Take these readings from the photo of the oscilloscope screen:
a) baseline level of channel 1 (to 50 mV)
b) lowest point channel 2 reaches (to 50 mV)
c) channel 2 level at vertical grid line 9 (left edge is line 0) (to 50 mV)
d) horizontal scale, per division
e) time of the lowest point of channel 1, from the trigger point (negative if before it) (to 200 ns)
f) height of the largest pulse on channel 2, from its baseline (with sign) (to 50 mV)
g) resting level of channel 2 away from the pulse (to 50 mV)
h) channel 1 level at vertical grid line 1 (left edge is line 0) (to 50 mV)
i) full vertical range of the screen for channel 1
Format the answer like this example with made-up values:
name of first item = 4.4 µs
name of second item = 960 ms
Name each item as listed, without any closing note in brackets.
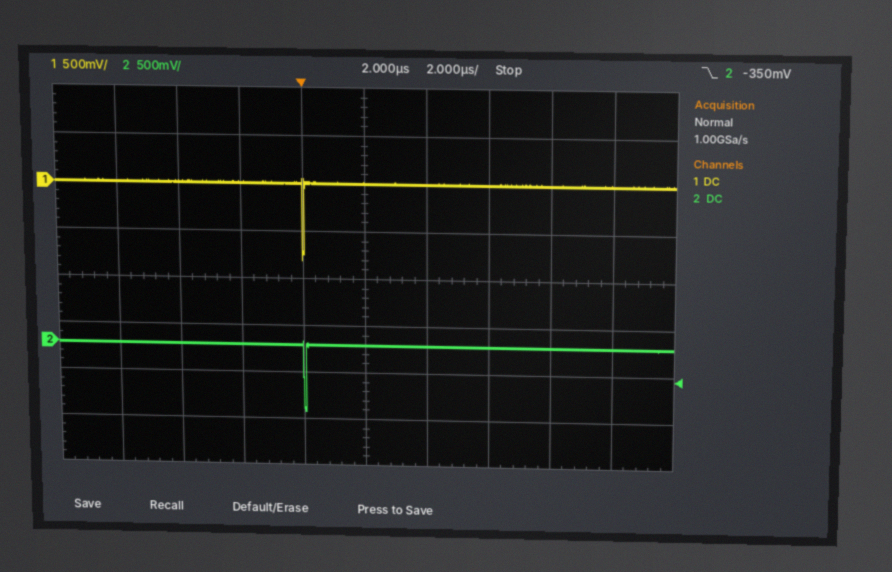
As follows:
baseline level of channel 1 = 0 mV
lowest point channel 2 reaches = -700 mV
channel 2 level at vertical grid line 9 (left edge is line 0) = 0 mV
horizontal scale, per division = 2 µs
time of the lowest point of channel 1, from the trigger point (negative if before it) = 0.0 µs
height of the largest pulse on channel 2, from its baseline (with sign) = -700 mV
resting level of channel 2 away from the pulse = 0 mV
channel 1 level at vertical grid line 1 (left edge is line 0) = 0 mV
full vertical range of the screen for channel 1 = 4 V
